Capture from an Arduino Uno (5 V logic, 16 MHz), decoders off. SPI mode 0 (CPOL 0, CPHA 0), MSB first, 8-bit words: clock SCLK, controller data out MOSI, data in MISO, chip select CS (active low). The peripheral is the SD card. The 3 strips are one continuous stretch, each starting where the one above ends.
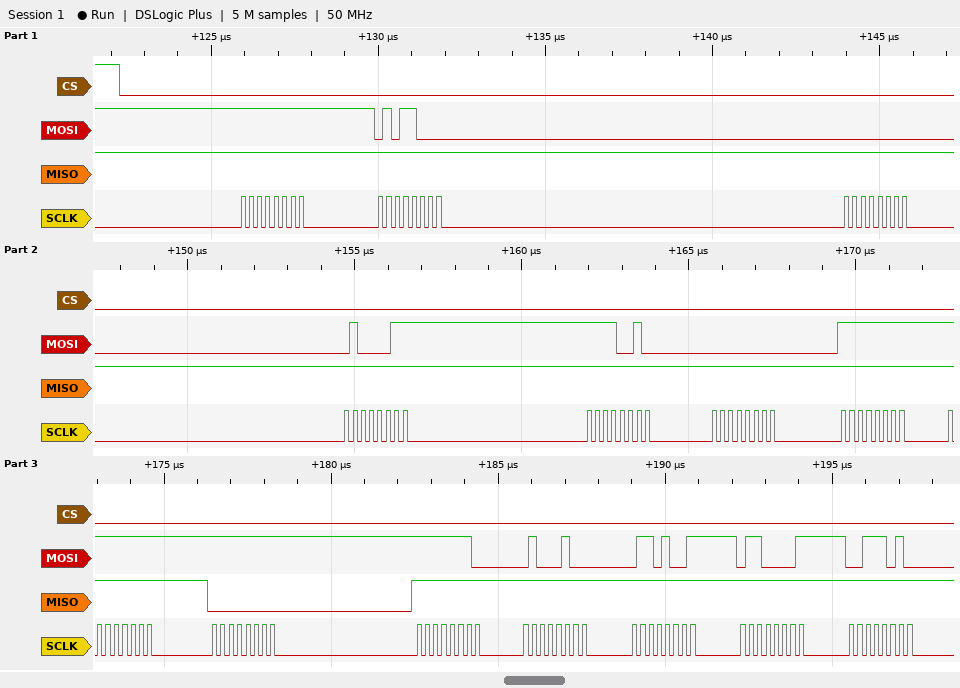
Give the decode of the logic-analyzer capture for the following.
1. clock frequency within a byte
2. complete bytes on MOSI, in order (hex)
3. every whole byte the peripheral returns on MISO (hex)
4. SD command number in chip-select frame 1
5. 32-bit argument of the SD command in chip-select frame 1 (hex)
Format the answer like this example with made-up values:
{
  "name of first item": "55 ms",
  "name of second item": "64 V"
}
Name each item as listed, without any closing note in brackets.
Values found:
{
  "clock frequency within a byte": "4 MHz",
  "complete bytes on MOSI, in order": "FF 58 00 43 F2 00 FF FF FF FE 44 69 61 3A",
  "every whole byte the peripheral returns on MISO": "FF FF FF FF FF FF FF FF 00 FF FF FF FF FF",
  "SD command number in chip-select frame 1": "CMD24",
  "32-bit argument of the SD command in chip-select frame 1": "0x0043F200"
}
